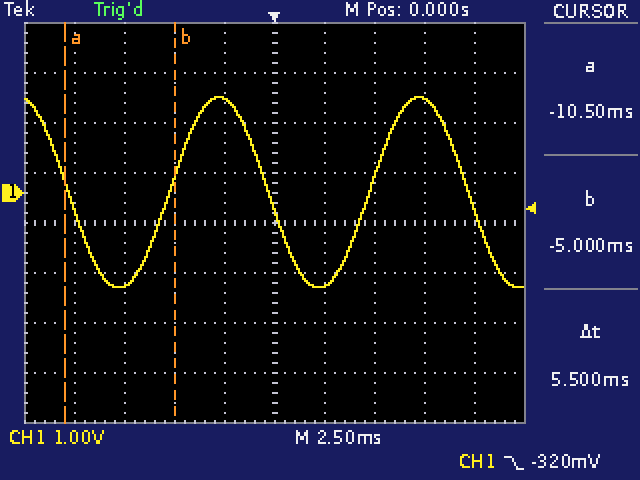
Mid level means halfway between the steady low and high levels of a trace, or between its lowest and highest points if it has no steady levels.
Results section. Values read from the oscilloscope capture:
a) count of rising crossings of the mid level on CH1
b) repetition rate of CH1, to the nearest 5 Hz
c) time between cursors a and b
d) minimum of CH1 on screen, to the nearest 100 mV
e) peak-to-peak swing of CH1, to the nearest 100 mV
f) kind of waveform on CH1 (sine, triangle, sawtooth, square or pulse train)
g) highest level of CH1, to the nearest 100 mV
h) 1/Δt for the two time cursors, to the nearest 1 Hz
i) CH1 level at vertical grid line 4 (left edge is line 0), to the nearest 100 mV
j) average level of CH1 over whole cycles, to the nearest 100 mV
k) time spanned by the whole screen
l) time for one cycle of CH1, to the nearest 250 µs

2
100 Hz
5.5 ms
-1.9 V
3.8 V
sine
1.9 V
182 Hz
1.9 V
0.0 V
25 ms
10.00 ms
